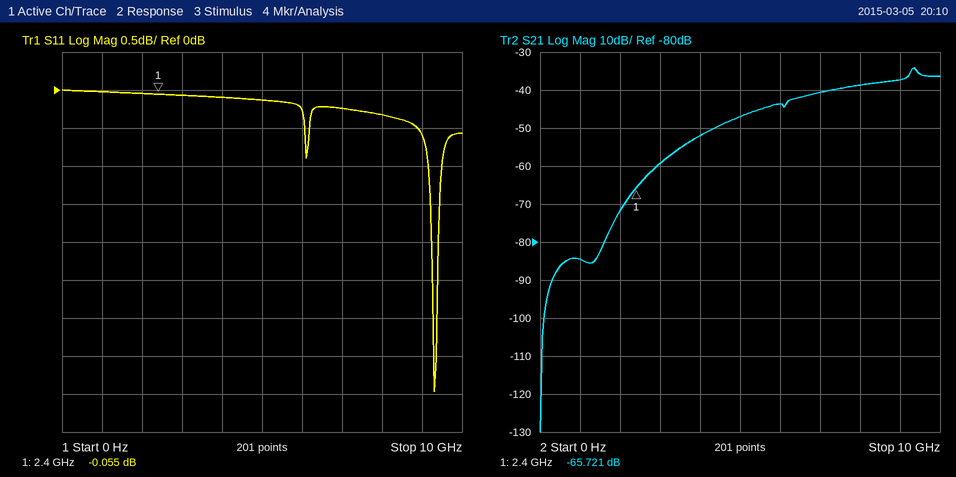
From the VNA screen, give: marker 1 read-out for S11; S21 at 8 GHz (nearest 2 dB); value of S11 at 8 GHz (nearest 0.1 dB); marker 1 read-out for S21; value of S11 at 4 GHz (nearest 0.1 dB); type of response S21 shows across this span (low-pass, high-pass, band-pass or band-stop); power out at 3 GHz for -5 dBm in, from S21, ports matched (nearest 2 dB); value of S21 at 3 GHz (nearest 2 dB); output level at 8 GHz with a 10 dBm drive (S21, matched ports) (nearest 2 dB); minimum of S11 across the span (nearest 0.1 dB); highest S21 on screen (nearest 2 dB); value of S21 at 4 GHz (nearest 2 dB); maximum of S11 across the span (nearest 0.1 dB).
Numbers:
-0.055 dB
-38 dB
-0.3 dB
-65.721 dB
-0.1 dB
high-pass
-64 dBm
-60 dB
-28 dBm
-4.0 dB
-34 dB
-52 dB
0.0 dB
